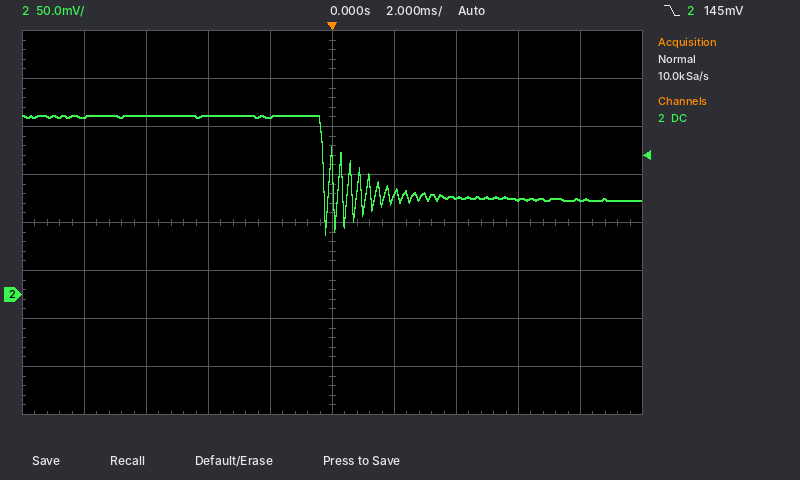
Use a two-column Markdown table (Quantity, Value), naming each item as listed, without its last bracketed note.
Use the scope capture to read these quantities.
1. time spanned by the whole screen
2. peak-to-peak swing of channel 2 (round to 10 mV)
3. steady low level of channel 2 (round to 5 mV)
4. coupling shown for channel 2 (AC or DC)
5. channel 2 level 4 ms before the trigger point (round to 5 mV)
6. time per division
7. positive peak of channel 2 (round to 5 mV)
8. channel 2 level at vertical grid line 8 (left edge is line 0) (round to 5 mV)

| Quantity | Value |
|---|---|
| time spanned by the whole screen | 20 ms |
| peak-to-peak swing of channel 2 | 120 mV |
| steady low level of channel 2 | 100 mV |
| coupling shown for channel 2 | DC |
| channel 2 level 4 ms before the trigger point | 185 mV |
| time per division | 2 ms |
| positive peak of channel 2 | 185 mV |
| channel 2 level at vertical grid line 8 (left edge is line 0) | 100 mV |
